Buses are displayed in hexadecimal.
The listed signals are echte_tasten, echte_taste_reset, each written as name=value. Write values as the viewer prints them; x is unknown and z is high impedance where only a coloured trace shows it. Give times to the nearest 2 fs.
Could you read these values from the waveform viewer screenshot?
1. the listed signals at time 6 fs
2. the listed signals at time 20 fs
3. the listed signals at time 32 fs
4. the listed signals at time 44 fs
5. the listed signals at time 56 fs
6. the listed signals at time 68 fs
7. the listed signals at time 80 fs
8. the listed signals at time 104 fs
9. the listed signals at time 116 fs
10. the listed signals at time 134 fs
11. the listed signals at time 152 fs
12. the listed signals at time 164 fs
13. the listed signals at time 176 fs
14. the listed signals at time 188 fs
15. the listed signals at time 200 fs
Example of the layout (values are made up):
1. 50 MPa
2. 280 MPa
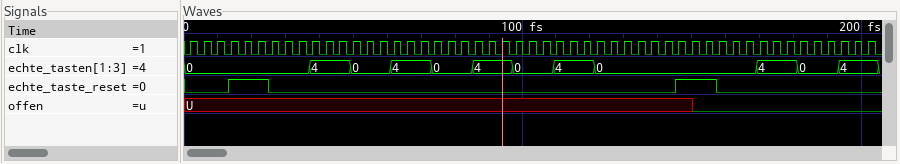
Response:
1. echte_tasten=0, echte_taste_reset=0
2. echte_tasten=0, echte_taste_reset=1
3. echte_tasten=0, echte_taste_reset=0
4. echte_tasten=4, echte_taste_reset=0
5. echte_tasten=0, echte_taste_reset=0
6. echte_tasten=4, echte_taste_reset=0
7. echte_tasten=0, echte_taste_reset=0
8. echte_tasten=0, echte_taste_reset=0
9. echte_tasten=4, echte_taste_reset=0
10. echte_tasten=0, echte_taste_reset=0
11. echte_tasten=0, echte_taste_reset=1
12. echte_tasten=0, echte_taste_reset=0
13. echte_tasten=4, echte_taste_reset=0
14. echte_tasten=0, echte_taste_reset=0
15. echte_tasten=4, echte_taste_reset=0
